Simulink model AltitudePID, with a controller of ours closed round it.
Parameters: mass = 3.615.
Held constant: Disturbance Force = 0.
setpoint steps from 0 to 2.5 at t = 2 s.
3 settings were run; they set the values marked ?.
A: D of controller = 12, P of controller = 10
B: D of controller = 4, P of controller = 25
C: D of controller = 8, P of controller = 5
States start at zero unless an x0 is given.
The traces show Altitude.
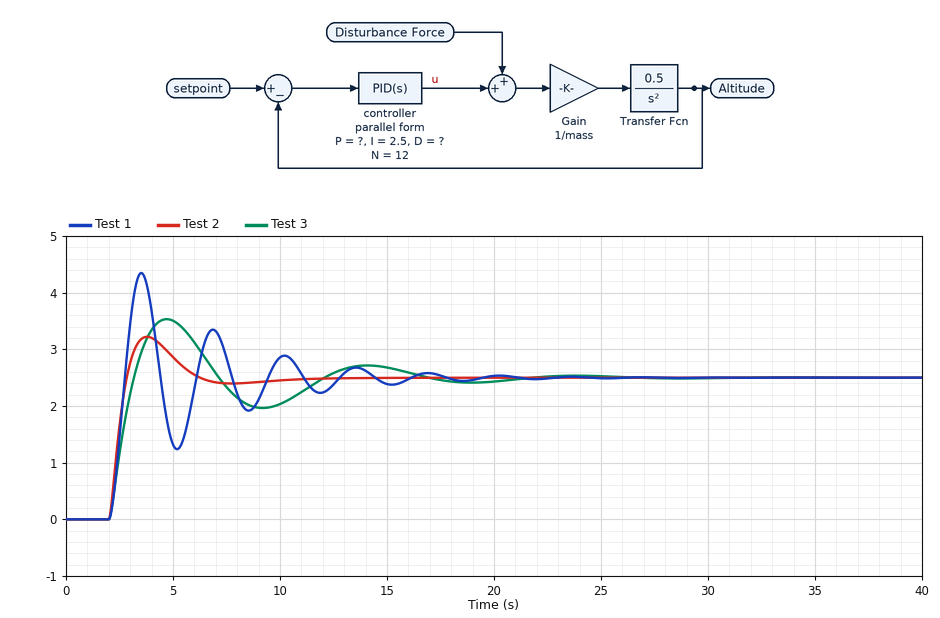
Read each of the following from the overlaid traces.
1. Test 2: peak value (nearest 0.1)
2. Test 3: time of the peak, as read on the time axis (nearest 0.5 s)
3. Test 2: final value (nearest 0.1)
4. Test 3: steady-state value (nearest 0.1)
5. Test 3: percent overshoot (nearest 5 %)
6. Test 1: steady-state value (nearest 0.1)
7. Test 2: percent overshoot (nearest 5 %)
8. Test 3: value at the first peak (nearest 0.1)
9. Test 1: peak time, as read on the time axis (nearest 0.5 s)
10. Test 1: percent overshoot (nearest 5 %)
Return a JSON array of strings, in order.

["3.2", "4.5 s", "2.5", "2.5", "40 %", "2.5", "30 %", "3.5", "3.5 s", "75 %"]
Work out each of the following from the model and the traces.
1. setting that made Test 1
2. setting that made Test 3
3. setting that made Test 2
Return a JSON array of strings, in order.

["B", "C", "A"]
